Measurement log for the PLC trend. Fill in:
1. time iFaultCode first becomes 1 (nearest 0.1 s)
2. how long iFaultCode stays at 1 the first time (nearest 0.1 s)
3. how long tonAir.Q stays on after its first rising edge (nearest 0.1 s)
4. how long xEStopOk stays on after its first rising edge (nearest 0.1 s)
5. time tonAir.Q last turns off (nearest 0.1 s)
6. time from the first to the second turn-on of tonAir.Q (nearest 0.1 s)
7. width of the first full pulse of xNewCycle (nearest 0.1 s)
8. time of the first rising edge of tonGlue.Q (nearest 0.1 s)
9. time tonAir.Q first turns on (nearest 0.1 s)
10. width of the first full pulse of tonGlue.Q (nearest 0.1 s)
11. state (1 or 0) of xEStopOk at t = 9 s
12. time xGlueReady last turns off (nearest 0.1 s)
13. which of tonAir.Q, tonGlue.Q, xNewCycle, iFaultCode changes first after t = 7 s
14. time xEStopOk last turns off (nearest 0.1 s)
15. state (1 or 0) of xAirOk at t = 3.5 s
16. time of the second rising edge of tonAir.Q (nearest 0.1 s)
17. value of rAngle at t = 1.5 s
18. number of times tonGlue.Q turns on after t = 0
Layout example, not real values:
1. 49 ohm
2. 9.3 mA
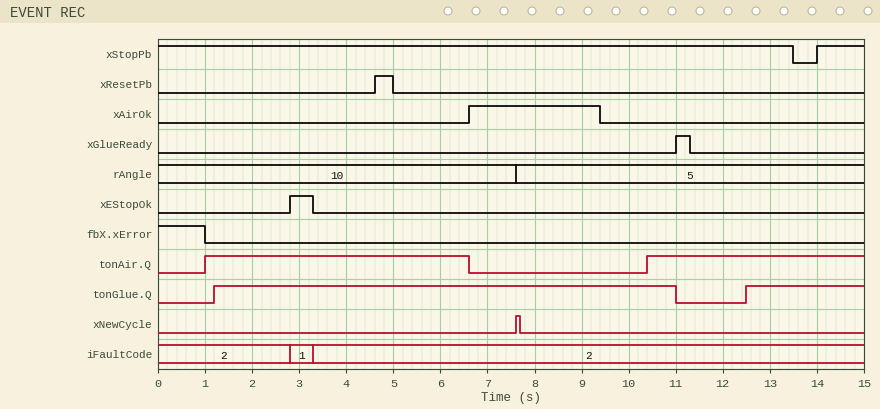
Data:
1. 2.8 s
2. 0.5 s
3. 5.6 s
4. 0.5 s
5. 6.6 s
6. 9.4 s
7. 0.1 s
8. 1.2 s
9. 1.0 s
10. 9.8 s
11. 0
12. 11.3 s
13. xNewCycle
14. 3.3 s
15. 0
16. 10.4 s
17. 10
18. 2
